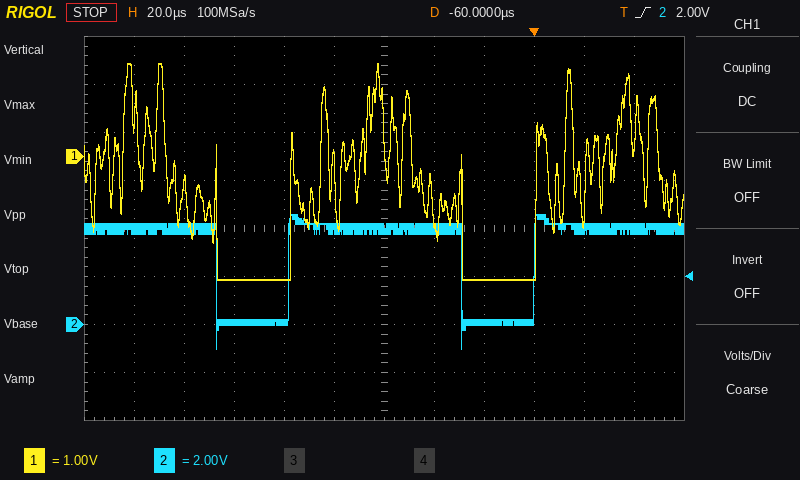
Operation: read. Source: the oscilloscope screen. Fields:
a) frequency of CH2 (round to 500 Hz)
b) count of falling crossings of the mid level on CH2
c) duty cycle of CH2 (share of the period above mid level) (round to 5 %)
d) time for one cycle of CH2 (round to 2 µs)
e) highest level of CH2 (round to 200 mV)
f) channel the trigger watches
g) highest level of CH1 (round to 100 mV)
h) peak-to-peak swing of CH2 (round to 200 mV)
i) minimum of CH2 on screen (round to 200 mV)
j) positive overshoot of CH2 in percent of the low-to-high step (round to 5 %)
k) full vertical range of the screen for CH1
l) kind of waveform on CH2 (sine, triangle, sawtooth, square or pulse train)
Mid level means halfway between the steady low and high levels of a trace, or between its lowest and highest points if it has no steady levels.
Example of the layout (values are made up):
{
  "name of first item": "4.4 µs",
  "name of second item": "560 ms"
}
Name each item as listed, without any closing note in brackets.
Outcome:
{
  "frequency of CH2": "10.0 kHz",
  "count of falling crossings of the mid level on CH2": "2",
  "duty cycle of CH2 (share of the period above mid level)": "70 %",
  "time for one cycle of CH2": "98 µs",
  "highest level of CH2": "4.6 V",
  "channel the trigger watches": "CH2",
  "highest level of CH1": "1.9 V",
  "peak-to-peak swing of CH2": "5.6 V",
  "minimum of CH2 on screen": "-1.0 V",
  "positive overshoot of CH2 in percent of the low-to-high step": "15 %",
  "full vertical range of the screen for CH1": "8 V",
  "kind of waveform on CH2": "pulse train"
}
